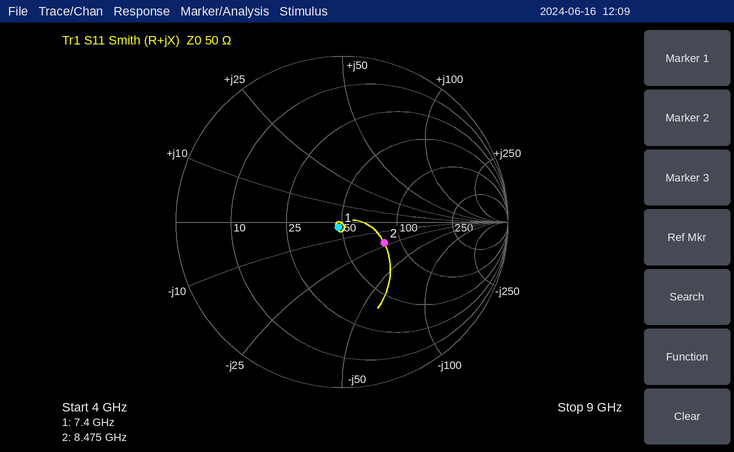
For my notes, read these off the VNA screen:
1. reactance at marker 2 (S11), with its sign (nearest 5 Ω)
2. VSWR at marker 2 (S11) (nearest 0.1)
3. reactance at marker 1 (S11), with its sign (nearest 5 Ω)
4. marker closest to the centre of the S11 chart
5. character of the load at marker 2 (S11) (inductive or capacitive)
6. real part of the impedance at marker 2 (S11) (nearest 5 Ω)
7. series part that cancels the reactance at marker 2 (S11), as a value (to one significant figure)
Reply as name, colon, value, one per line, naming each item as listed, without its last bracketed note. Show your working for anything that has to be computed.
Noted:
reactance at marker 2 (S11), with its sign: -20 Ω
VSWR at marker 2 (S11): 1.8
reactance at marker 1 (S11), with its sign: -5 Ω
marker closest to the centre of the S11 chart: marker 1
character of the load at marker 2 (S11): capacitive
real part of the impedance at marker 2 (S11): 80 Ω
series part that cancels the reactance at marker 2 (S11), as a value: L = 20 Ω/(2π × 8.475 GHz) ≈ 376 pH, so 400 pH to one significant figure
